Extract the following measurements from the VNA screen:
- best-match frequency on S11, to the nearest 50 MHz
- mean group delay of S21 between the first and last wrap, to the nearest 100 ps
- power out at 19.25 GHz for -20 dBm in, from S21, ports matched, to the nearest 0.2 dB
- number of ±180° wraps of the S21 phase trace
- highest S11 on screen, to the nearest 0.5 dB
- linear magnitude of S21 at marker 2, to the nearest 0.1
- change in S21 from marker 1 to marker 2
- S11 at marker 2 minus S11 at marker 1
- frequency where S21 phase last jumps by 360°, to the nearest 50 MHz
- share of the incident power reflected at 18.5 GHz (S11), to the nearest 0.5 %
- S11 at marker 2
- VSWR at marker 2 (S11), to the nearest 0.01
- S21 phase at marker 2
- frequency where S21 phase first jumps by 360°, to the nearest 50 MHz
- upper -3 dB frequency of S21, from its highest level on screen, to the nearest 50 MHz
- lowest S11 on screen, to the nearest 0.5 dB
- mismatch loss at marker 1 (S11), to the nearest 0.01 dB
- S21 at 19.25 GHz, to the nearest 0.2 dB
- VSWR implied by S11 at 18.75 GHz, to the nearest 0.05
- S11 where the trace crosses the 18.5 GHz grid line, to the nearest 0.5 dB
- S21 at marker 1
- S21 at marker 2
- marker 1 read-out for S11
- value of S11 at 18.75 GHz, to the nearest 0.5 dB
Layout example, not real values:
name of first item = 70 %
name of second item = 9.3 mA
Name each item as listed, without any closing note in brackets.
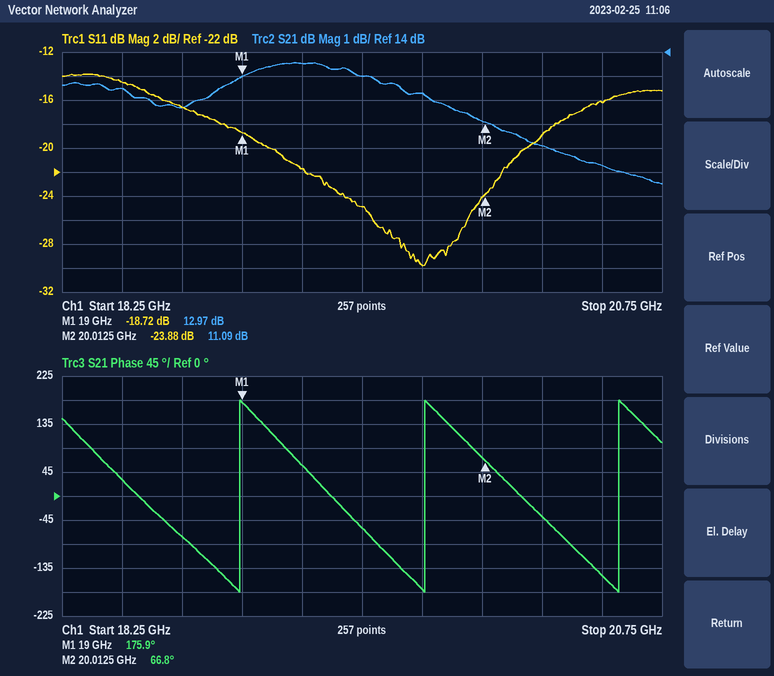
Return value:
best-match frequency on S11, to the nearest 50 MHz = 19.75 GHz
mean group delay of S21 between the first and last wrap, to the nearest 100 ps = 1.3 ns
power out at 19.25 GHz for -20 dBm in, from S21, ports matched, to the nearest 0.2 dB = -6.4 dBm
number of ±180° wraps of the S21 phase trace = 3
highest S11 on screen, to the nearest 0.5 dB = -14.0 dB
linear magnitude of S21 at marker 2, to the nearest 0.1 = 3.6
change in S21 from marker 1 to marker 2 = -1.88 dB
S11 at marker 2 minus S11 at marker 1 = -5.16 dB
frequency where S21 phase last jumps by 360°, to the nearest 50 MHz = 20.55 GHz
share of the incident power reflected at 18.5 GHz (S11), to the nearest 0.5 % = 3.5 %
S11 at marker 2 = -23.88 dB
VSWR at marker 2 (S11), to the nearest 0.01 = 1.14
S21 phase at marker 2 = 66.8°
frequency where S21 phase first jumps by 360°, to the nearest 50 MHz = 19.00 GHz
upper -3 dB frequency of S21, from its highest level on screen, to the nearest 50 MHz = 20.15 GHz
lowest S11 on screen, to the nearest 0.5 dB = -30.0 dB
mismatch loss at marker 1 (S11), to the nearest 0.01 dB = 0.06 dB
S21 at 19.25 GHz, to the nearest 0.2 dB = 13.6 dB
VSWR implied by S11 at 18.75 GHz, to the nearest 0.05 = 1.35
S11 where the trace crosses the 18.5 GHz grid line, to the nearest 0.5 dB = -14.5 dB
S21 at marker 1 = 12.97 dB
S21 at marker 2 = 11.09 dB
marker 1 read-out for S11 = -18.72 dB
value of S11 at 18.75 GHz, to the nearest 0.5 dB = -16.5 dB
